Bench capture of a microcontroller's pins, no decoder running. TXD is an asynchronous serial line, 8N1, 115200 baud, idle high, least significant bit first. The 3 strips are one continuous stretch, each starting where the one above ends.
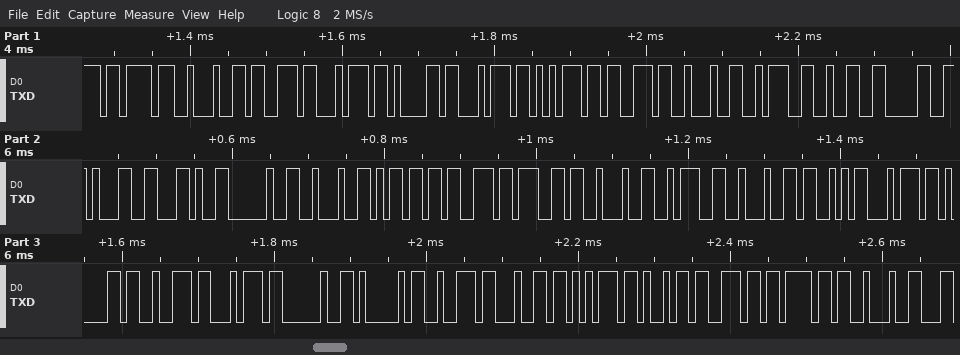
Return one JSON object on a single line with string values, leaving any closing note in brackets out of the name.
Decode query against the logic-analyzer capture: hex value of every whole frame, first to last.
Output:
{"hex value of every whole frame, first to last": "7B 22 73 74 61 74 75 73 22 3A 32 30 31 2C 20 22 6D 73 67 22 3A 22 53 74 61 72 74 20 41 72 64 75 69 6E 6F 22"}
